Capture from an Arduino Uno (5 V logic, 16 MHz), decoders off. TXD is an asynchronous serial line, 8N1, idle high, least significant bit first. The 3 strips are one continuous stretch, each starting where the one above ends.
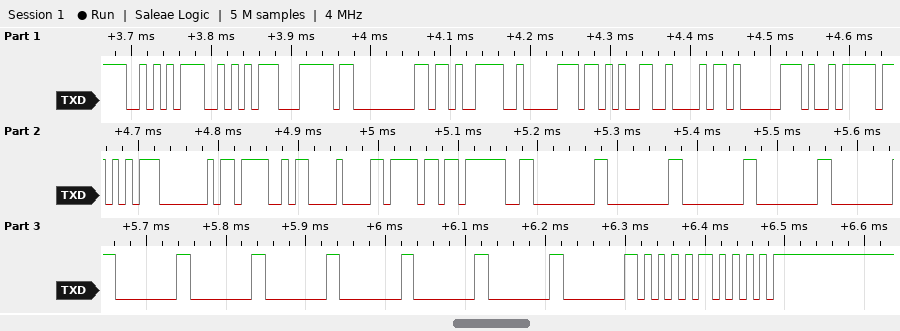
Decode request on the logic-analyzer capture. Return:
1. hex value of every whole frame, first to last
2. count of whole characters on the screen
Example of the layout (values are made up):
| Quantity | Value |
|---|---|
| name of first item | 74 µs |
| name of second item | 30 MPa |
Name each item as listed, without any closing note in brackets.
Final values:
| Quantity | Value |
|---|---|
| hex value of every whole frame, first to last | AA AA 7C 00 CB 82 2B 42 81 E9 AB 40 4F 08 6F 3F 00 00 00 00 00 00 00 00 00 00 00 00 55 55 |
| count of whole characters on the screen | 30 |
